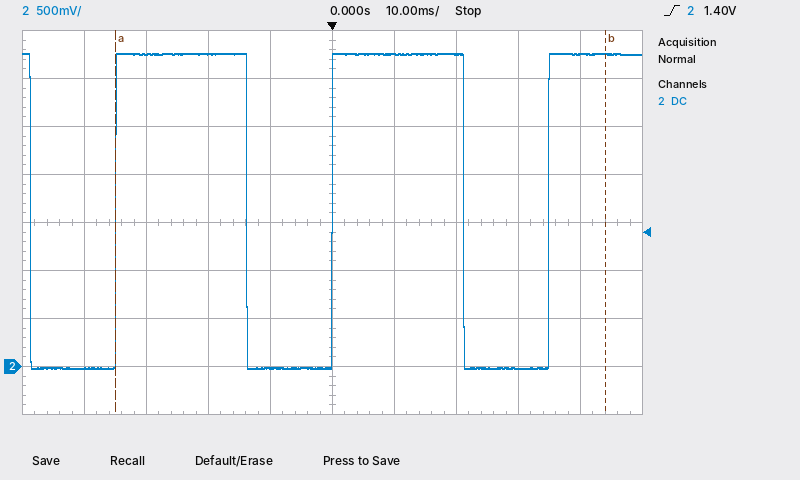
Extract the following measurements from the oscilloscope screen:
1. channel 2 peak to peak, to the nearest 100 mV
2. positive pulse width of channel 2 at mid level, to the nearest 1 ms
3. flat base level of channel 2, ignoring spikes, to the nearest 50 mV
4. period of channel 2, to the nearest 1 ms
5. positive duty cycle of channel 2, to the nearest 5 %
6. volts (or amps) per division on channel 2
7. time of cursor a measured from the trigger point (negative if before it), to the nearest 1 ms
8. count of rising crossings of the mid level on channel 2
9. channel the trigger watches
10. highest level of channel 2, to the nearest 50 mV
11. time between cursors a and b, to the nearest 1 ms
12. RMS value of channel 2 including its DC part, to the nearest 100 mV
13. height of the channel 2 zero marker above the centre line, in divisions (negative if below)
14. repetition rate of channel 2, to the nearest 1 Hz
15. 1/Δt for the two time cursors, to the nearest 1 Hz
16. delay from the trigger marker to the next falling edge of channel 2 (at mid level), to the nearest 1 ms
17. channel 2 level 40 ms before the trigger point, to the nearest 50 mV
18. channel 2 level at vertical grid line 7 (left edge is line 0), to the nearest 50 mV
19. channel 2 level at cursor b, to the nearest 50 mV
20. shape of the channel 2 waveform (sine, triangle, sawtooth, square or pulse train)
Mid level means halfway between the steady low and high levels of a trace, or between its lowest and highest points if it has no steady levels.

3.30 V
21 ms
0 mV
35 ms
60 %
500 mV
-35 ms
3
channel 2
3.25 V
79 ms
2.5 V
-3.0 div
29 Hz
13 Hz
21 ms
0 mV
3.25 V
3.25 V
pulse train
